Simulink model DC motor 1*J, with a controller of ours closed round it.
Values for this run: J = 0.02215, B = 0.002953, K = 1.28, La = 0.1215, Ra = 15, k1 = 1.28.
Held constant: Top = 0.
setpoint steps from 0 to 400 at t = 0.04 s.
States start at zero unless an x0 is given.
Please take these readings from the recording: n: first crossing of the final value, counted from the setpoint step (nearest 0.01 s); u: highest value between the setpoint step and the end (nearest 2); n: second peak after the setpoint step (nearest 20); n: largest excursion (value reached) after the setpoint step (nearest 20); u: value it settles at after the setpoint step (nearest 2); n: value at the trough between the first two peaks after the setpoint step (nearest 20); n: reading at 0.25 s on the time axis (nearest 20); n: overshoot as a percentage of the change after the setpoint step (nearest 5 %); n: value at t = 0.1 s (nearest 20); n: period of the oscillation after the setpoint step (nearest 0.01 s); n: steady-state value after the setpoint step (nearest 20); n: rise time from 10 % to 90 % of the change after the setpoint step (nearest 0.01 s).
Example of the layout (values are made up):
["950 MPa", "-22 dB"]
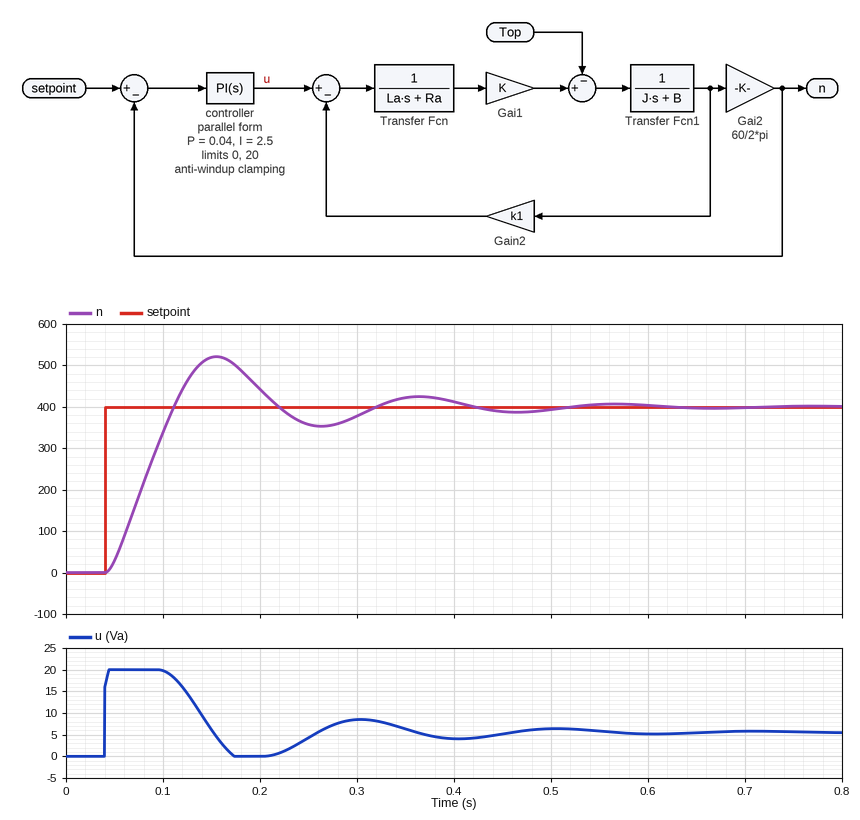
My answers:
["0.07 s", "20", "420", "520", "6", "360", "360", "30 %", "340", "0.21 s", "400", "0.05 s"]
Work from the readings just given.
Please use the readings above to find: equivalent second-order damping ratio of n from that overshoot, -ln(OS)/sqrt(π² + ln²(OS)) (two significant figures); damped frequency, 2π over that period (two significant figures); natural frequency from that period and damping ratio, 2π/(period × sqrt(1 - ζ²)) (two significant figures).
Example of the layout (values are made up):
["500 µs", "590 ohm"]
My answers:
["0.36", "30 rad/s", "32 rad/s"]
